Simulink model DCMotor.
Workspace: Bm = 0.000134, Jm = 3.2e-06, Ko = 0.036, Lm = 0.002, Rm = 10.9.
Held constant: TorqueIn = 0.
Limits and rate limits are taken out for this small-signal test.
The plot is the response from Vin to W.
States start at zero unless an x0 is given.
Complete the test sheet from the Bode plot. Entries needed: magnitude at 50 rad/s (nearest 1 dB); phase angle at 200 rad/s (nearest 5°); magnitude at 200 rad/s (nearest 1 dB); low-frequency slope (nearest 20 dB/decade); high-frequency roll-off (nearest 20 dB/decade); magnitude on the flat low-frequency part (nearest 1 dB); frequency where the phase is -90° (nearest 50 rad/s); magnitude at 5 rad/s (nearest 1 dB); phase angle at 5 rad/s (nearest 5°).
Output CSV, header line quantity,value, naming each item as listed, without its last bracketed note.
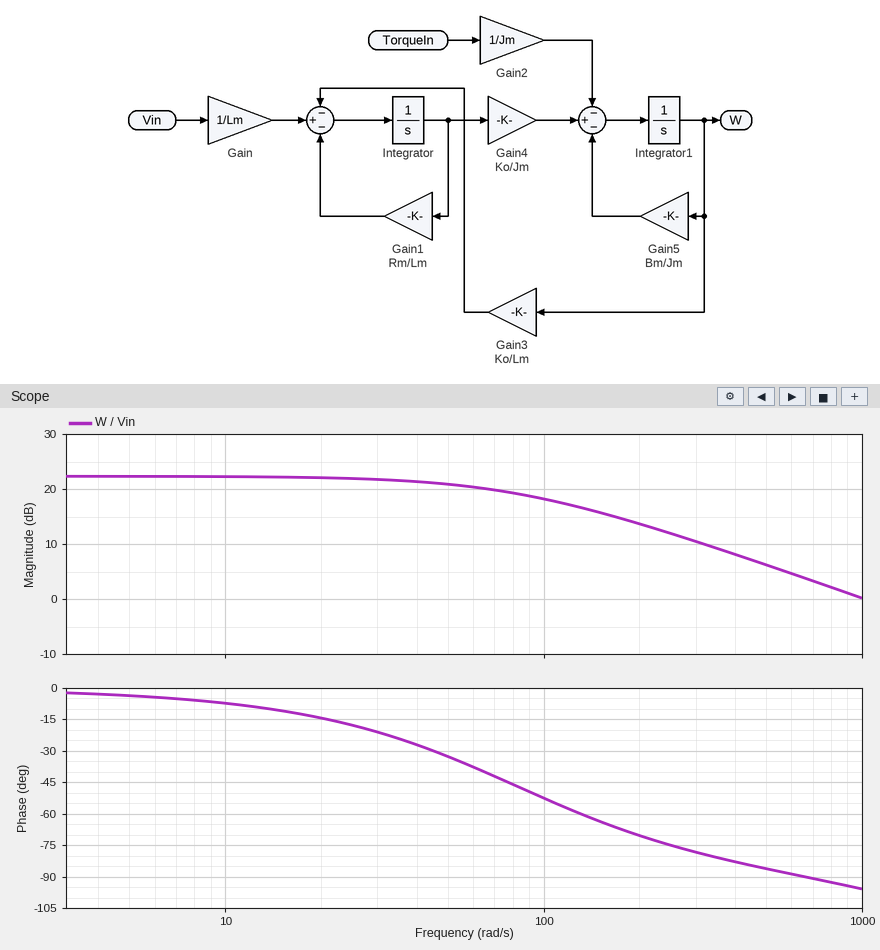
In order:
quantity,value
magnitude at 50 rad/s,21 dB
phase angle at 200 rad/s,-70°
magnitude at 200 rad/s,14 dB
low-frequency slope,0 dB/decade
high-frequency roll-off,-20 dB/decade
magnitude on the flat low-frequency part,22 dB
frequency where the phase is -90°,650 rad/s
magnitude at 5 rad/s,22 dB
phase angle at 5 rad/s,-5°
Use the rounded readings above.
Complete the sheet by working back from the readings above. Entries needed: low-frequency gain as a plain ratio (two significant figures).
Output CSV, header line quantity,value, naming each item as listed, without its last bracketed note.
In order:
quantity,value
low-frequency gain as a plain ratio,13
